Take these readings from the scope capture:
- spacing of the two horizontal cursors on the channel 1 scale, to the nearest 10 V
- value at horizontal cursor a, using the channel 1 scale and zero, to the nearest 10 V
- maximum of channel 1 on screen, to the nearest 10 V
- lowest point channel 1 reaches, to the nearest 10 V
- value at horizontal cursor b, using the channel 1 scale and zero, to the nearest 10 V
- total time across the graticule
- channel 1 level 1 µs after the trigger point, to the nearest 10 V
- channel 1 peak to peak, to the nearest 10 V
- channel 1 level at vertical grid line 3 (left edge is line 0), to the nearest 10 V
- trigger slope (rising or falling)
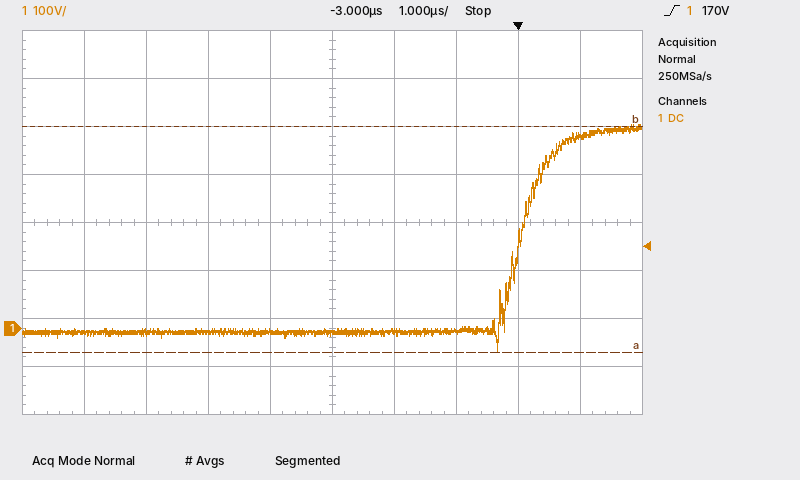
470 V
-50 V
420 V
-50 V
420 V
10 µs
400 V
470 V
-10 V
rising
